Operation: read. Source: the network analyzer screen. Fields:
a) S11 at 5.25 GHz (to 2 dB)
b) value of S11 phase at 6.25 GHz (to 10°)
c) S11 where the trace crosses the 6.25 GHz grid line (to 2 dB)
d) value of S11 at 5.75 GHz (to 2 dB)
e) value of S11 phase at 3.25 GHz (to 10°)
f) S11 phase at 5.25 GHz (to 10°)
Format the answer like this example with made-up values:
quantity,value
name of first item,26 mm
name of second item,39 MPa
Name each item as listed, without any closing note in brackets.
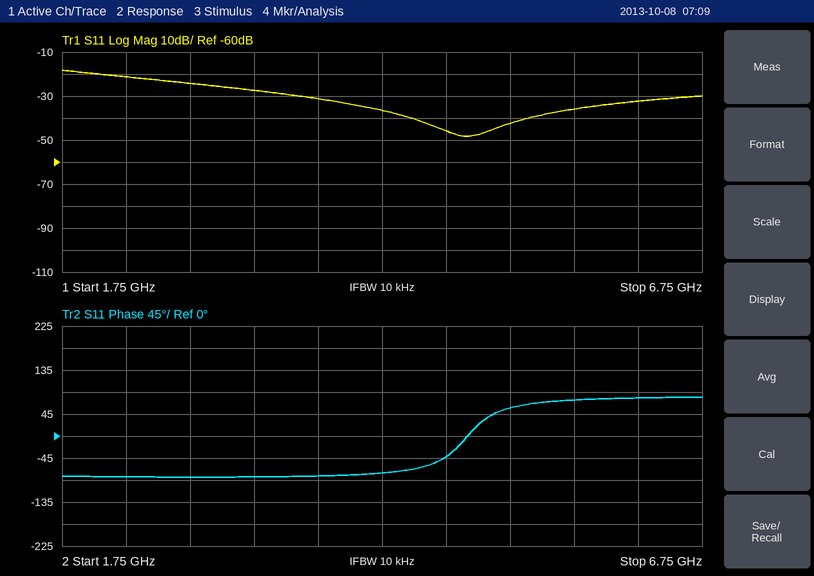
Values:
quantity,value
S11 at 5.25 GHz,-42 dB
value of S11 phase at 6.25 GHz,80°
S11 where the trace crosses the 6.25 GHz grid line,-32 dB
value of S11 at 5.75 GHz,-36 dB
value of S11 phase at 3.25 GHz,-80°
S11 phase at 5.25 GHz,60°
